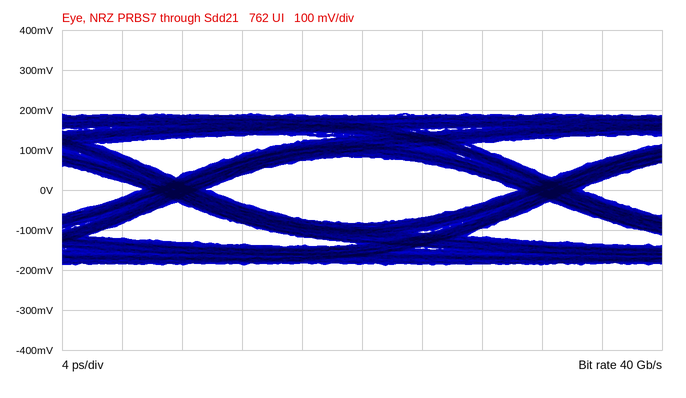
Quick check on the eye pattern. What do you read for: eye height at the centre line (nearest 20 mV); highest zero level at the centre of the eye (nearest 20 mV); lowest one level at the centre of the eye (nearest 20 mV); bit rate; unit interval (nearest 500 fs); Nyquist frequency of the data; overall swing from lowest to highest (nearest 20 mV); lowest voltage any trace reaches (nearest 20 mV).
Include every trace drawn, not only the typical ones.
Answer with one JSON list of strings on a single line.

["160 mV", "-80 mV", "80 mV", "40 Gb/s", "25.0 ps", "20 GHz", "380 mV", "-180 mV"]
